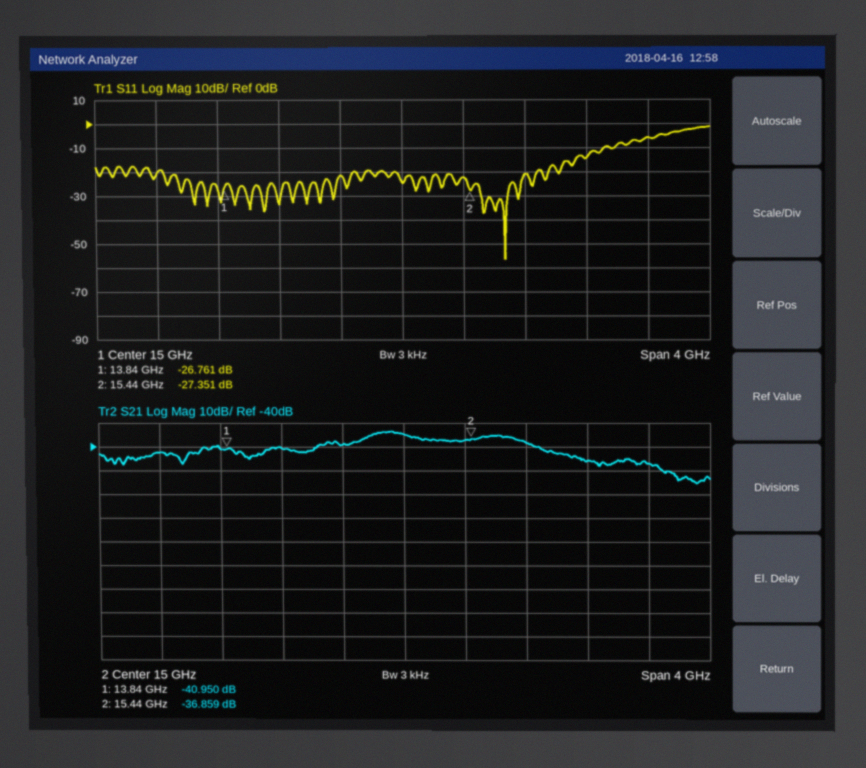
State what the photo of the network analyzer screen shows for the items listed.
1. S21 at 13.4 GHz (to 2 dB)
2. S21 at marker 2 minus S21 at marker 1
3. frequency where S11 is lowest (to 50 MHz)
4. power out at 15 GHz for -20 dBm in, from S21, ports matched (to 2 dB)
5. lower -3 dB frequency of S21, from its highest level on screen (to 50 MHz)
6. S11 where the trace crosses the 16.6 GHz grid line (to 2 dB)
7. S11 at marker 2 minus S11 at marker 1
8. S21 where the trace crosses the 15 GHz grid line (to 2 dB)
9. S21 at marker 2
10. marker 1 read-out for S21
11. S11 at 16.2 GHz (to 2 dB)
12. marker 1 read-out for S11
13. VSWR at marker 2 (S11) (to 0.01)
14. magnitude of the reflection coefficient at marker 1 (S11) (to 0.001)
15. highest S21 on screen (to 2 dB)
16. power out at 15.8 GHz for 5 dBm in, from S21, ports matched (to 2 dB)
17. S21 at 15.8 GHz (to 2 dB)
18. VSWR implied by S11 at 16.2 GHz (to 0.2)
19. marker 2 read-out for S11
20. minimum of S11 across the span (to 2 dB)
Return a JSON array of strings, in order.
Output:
["-42 dB", "4.091 dB", "15.65 GHz", "-54 dBm", "14.75 GHz", "-6 dB", "-0.590 dB", "-34 dB", "-36.859 dB", "-40.950 dB", "-14 dB", "-26.761 dB", "1.09", "0.046", "-34 dB", "-34 dBm", "-38 dB", "1.4", "-27.351 dB", "-56 dB"]
